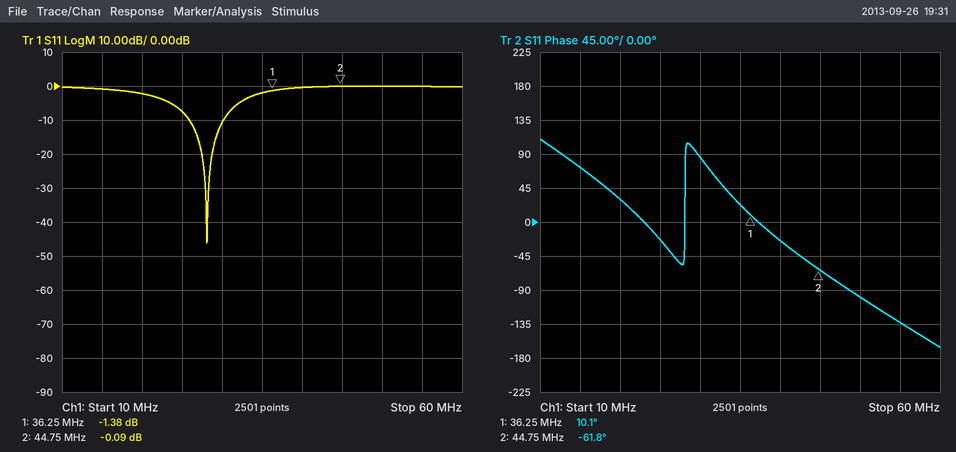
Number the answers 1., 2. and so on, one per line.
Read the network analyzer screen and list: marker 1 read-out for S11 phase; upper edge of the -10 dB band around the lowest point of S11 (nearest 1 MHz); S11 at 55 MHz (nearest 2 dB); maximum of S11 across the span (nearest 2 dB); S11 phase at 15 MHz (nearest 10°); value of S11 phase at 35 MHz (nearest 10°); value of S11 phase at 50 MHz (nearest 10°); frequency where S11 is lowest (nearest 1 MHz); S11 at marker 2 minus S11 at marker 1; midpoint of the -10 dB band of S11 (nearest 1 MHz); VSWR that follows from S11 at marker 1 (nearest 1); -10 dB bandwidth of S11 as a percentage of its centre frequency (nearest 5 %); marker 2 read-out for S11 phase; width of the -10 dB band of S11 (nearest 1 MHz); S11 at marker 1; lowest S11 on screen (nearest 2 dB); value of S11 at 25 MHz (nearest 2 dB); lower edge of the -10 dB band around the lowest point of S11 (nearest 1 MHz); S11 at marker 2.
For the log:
1. 10.1°
2. 30 MHz
3. 0 dB
4. 0 dB
5. 70°
6. 20°
7. -100°
8. 28 MHz
9. 1.29 dB
10. 28 MHz
11. 13
12. 15 %
13. -61.8°
14. 4 MHz
15. -1.38 dB
16. -46 dB
17. -8 dB
18. 26 MHz
19. -0.09 dB
